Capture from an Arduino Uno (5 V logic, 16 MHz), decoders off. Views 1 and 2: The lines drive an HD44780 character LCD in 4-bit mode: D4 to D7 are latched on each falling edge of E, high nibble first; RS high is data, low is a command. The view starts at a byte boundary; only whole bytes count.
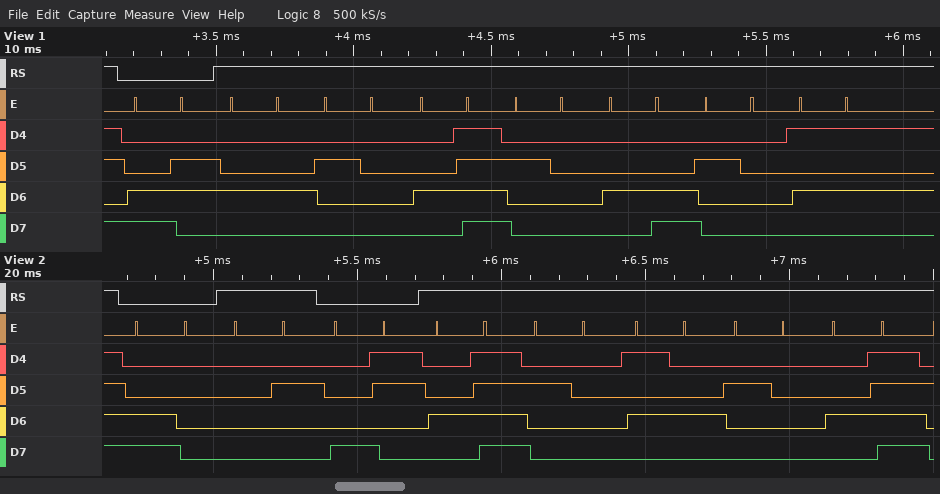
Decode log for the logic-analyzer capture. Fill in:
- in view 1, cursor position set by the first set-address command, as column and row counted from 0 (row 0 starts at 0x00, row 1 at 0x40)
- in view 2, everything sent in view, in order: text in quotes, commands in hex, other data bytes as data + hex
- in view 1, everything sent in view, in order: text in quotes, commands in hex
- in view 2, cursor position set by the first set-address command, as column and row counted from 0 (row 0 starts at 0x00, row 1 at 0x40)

column 6, row 1
0xC0 data 02 0x83 "O T O"
0xC6 "D O L U"
column 0, row 1
